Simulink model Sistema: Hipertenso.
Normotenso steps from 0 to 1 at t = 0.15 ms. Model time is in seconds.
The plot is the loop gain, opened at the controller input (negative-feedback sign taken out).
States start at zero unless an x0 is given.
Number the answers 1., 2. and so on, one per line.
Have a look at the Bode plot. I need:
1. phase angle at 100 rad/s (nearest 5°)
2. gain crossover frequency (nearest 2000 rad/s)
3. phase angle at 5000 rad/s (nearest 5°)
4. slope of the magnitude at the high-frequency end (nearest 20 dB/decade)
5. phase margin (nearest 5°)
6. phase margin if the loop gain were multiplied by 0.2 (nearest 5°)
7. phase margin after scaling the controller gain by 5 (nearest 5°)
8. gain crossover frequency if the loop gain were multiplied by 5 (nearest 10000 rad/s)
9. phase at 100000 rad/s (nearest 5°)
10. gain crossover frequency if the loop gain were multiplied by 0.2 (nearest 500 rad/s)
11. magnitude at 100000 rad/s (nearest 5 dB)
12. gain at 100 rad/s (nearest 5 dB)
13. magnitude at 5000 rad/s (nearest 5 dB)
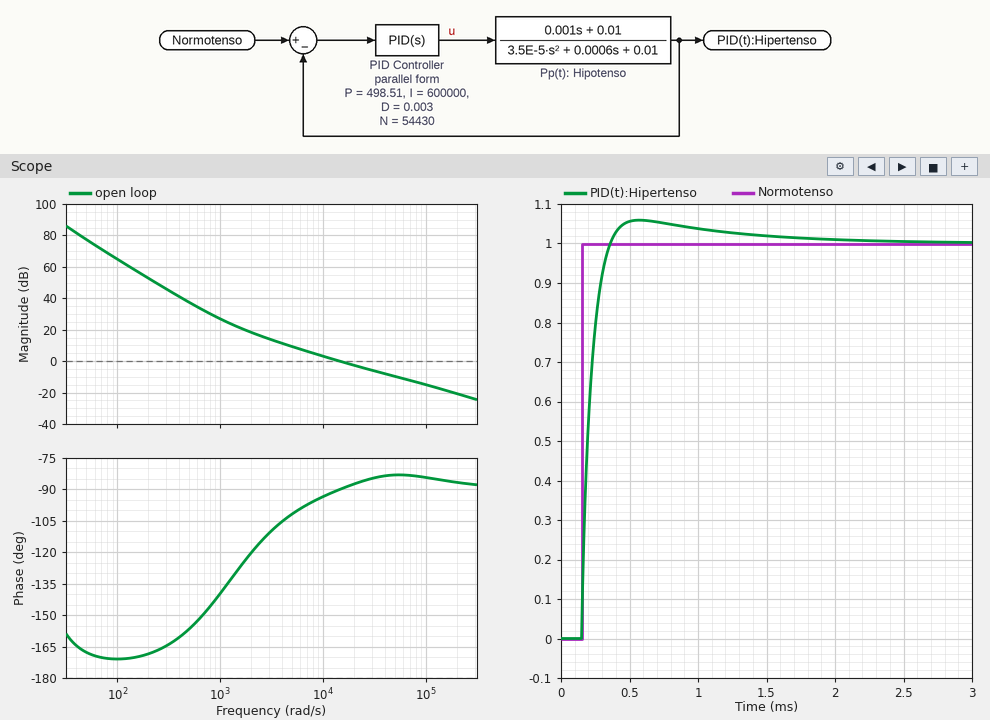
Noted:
1. -170°
2. 14000 rad/s
3. -100°
4. -20 dB/decade
5. 90°
6. 70°
7. 95°
8. 90000 rad/s
9. -85°
10. 3000 rad/s
11. -15 dB
12. 65 dB
13. 10 dB
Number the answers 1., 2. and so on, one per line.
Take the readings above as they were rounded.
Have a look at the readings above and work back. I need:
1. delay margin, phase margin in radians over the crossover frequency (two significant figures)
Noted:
1. 0.00011 s
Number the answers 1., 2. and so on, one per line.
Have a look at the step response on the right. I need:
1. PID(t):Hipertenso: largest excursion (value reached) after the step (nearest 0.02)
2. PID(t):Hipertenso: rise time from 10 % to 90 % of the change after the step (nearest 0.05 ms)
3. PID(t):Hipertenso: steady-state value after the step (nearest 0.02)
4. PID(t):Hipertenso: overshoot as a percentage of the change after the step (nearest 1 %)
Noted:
1. 1.06
2. 0.15 ms
3. 1.00
4. 6 %
